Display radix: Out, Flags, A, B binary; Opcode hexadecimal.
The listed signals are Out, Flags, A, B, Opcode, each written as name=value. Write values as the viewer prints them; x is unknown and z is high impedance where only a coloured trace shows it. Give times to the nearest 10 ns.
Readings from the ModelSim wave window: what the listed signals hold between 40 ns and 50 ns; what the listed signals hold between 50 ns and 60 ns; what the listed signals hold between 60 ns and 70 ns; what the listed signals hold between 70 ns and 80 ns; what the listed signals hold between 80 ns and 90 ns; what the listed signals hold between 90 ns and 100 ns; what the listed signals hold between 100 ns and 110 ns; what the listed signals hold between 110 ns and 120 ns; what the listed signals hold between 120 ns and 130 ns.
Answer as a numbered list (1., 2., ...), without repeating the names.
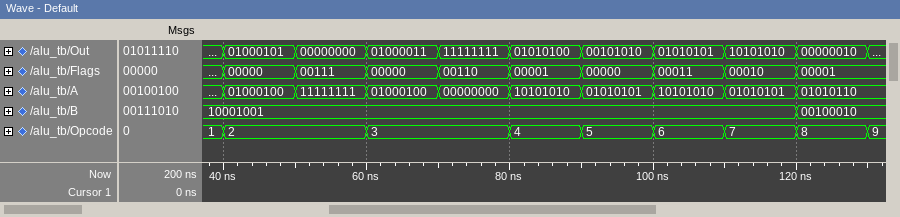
1. Out=01000101, Flags=00000, A=01000100, B=10001001, Opcode=2
2. Out=00000000, Flags=00111, A=11111111, B=10001001, Opcode=2
3. Out=01000011, Flags=00000, A=01000100, B=10001001, Opcode=3
4. Out=11111111, Flags=00110, A=00000000, B=10001001, Opcode=3
5. Out=01010100, Flags=00001, A=10101010, B=10001001, Opcode=4
6. Out=00101010, Flags=00000, A=01010101, B=10001001, Opcode=5
7. Out=01010101, Flags=00011, A=10101010, B=10001001, Opcode=6
8. Out=10101010, Flags=00010, A=01010101, B=10001001, Opcode=7
9. Out=00000010, Flags=00001, A=01010110, B=00100010, Opcode=8
